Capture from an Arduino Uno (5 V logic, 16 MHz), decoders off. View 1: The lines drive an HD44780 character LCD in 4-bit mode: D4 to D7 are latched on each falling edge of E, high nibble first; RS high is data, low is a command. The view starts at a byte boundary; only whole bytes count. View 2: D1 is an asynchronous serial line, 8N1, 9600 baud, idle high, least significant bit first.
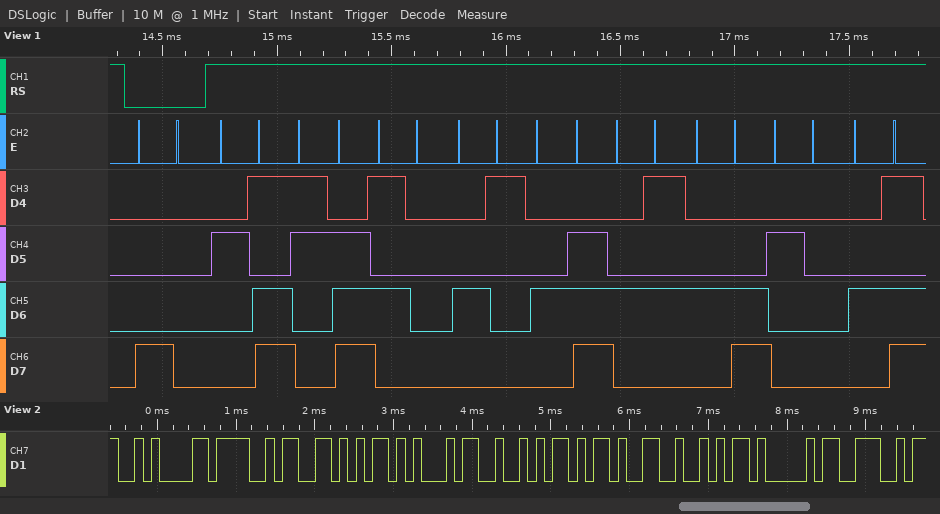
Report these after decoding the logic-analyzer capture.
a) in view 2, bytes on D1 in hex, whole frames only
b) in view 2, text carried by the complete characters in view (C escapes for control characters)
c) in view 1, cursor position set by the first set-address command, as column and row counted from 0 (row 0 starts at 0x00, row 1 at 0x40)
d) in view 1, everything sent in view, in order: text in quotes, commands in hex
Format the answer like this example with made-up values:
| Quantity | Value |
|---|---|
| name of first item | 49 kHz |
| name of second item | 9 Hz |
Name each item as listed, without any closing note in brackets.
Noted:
| Quantity | Value |
|---|---|
| in view 2, bytes on D1 in hex, whole frames only | 0x0A 0x4F 0x56 0x45 0x52 0x2D 0x52 0x41 0x4E |
| in view 2, text carried by the complete characters in view | "\nOVER-RAN" |
| in view 1, cursor position set by the first set-address command, as column and row counted from 0 | column 0, row 0 |
| in view 1, everything sent in view, in order: text in quotes, commands in hex | 0x80 "->PANEL M" |
